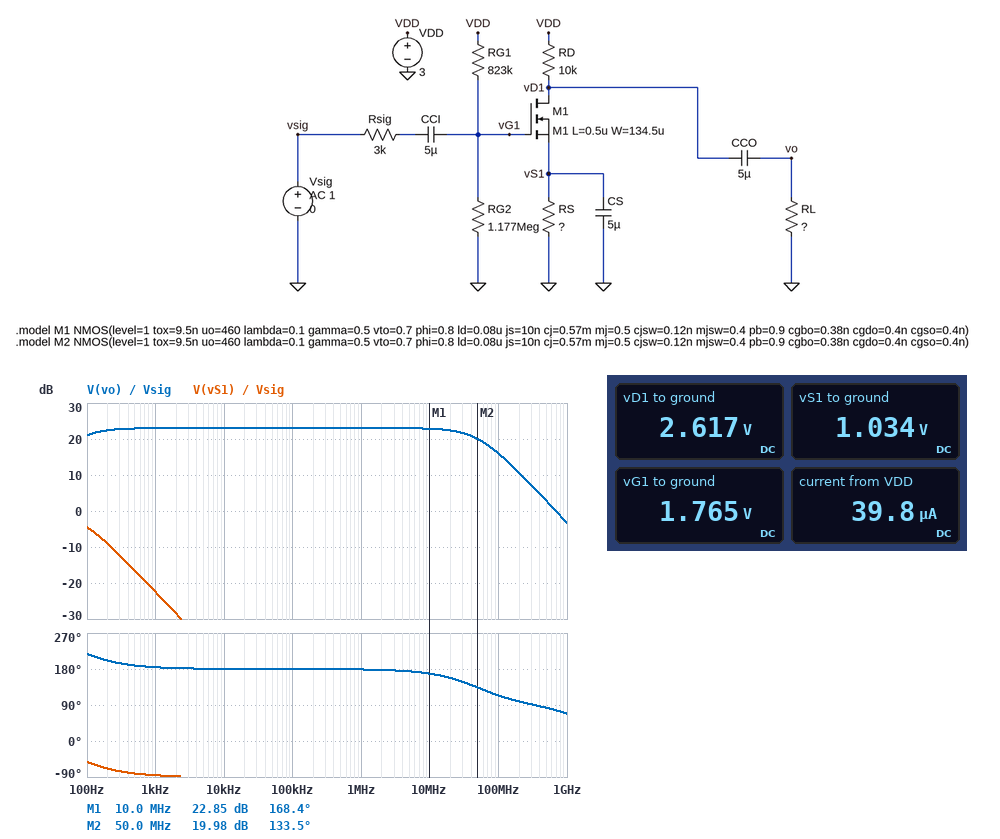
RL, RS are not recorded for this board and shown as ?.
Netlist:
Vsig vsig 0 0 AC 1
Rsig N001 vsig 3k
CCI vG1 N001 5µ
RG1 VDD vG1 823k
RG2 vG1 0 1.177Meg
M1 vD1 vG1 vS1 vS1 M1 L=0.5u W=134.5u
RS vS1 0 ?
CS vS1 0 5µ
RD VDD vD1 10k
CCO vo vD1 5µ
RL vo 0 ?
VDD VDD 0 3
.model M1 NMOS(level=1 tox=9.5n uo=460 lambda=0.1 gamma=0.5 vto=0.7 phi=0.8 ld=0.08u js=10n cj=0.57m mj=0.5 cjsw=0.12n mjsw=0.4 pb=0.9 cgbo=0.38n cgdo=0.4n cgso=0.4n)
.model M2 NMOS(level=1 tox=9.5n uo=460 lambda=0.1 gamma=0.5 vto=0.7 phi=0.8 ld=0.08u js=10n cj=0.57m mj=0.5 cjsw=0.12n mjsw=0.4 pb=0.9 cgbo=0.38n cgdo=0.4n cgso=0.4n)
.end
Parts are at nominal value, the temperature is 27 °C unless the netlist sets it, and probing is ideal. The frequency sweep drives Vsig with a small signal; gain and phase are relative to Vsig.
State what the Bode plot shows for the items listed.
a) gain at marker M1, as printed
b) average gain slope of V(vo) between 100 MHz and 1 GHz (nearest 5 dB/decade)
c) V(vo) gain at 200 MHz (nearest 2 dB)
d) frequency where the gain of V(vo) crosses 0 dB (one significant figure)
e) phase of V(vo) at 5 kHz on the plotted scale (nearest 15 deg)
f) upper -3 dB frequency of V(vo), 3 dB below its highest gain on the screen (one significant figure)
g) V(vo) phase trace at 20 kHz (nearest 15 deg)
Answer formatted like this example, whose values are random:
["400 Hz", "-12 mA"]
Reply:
["22.85 dB", "-20 dB/decade", "10 dB", "700 MHz", "180 deg", "50 MHz", "180 deg"]
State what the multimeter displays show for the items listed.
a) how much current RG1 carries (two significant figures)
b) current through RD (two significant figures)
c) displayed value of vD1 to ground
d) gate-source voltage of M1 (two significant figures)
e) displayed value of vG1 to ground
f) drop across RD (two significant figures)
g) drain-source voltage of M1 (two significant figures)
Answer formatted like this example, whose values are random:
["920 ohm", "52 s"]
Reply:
["1.5 µA", "38 µA", "2.617 V", "730 mV", "1.765 V", "380 mV", "1.6 V"]
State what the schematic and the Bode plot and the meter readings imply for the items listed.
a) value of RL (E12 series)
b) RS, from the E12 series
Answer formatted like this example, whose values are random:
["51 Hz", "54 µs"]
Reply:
["15 kΩ", "27 kΩ"]
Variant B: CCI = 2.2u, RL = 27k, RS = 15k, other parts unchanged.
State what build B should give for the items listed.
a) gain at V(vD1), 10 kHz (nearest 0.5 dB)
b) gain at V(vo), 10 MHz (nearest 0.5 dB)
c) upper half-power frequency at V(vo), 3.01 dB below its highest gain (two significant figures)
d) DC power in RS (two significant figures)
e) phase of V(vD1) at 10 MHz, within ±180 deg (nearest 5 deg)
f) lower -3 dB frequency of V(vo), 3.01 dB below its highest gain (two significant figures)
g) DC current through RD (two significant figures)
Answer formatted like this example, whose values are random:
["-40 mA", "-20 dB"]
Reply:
["27.0 dB", "26.5 dB", "35 MHz", "70 µW", "165 deg", "100 Hz", "68 µA"]
